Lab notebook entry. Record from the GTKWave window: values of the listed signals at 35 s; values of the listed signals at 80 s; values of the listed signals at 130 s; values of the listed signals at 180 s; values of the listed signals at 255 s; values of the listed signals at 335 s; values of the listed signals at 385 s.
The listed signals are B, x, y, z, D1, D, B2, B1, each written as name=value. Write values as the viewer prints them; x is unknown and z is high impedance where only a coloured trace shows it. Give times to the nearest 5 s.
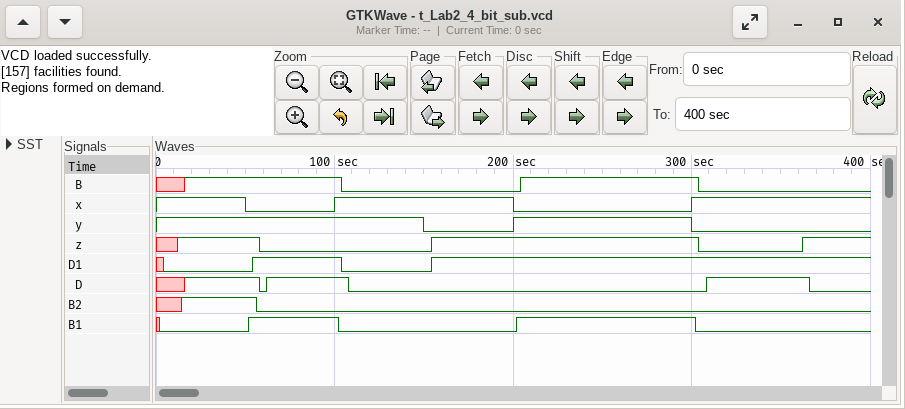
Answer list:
B=1, x=1, y=1, z=1, D1=0, D=1, B2=1, B1=0
B=1, x=0, y=1, z=0, D1=1, D=1, B2=0, B1=1
B=0, x=1, y=1, z=0, D1=0, D=0, B2=0, B1=0
B=0, x=1, y=0, z=1, D1=1, D=0, B2=0, B1=0
B=1, x=0, y=1, z=1, D1=1, D=0, B2=0, B1=1
B=0, x=1, y=0, z=0, D1=1, D=1, B2=0, B1=0
B=0, x=1, y=0, z=1, D1=1, D=0, B2=0, B1=0
